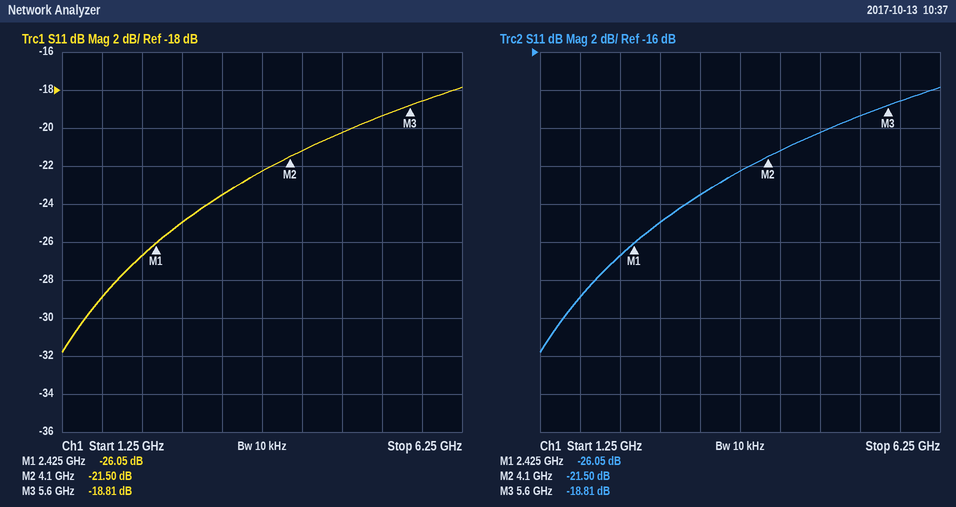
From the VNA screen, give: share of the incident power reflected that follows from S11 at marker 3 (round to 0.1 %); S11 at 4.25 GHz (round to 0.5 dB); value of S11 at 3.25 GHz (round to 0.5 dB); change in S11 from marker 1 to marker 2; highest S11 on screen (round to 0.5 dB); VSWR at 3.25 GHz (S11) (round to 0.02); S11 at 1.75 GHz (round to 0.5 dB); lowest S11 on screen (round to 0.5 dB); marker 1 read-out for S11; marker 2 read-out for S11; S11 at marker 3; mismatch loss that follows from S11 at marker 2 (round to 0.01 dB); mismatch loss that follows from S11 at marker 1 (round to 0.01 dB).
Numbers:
1.3 %
-21.0 dB
-23.5 dB
4.55 dB
-18.0 dB
1.14
-29.0 dB
-32.0 dB
-26.05 dB
-21.50 dB
-18.81 dB
0.03 dB
0.01 dB
